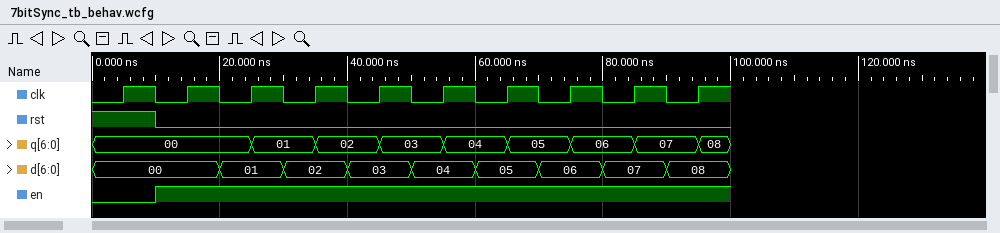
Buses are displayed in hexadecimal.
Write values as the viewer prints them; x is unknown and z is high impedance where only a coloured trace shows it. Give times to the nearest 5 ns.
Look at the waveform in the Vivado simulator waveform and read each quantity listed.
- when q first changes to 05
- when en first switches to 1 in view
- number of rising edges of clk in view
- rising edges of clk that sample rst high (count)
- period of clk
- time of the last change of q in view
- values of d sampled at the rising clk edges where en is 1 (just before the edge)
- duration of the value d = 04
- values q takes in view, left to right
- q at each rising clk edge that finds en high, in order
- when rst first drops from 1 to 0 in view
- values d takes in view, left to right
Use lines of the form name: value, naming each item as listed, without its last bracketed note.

when q first changes to 05: 65 ns
when en first switches to 1 in view: 10 ns
number of rising edges of clk in view: 10
rising edges of clk that sample rst high: 1
period of clk: 10 ns
time of the last change of q in view: 95 ns
values of d sampled at the rising clk edges where en is 1: 00, 01, 02, 03, 04, 05, 06, 07, 08
duration of the value d = 04: 10 ns
values q takes in view, left to right: 00, 01, 02, 03, 04, 05, 06, 07, 08
q at each rising clk edge that finds en high, in order: 00, 00, 01, 02, 03, 04, 05, 06, 07
when rst first drops from 1 to 0 in view: 10 ns
values d takes in view, left to right: 00, 01, 02, 03, 04, 05, 06, 07, 08
